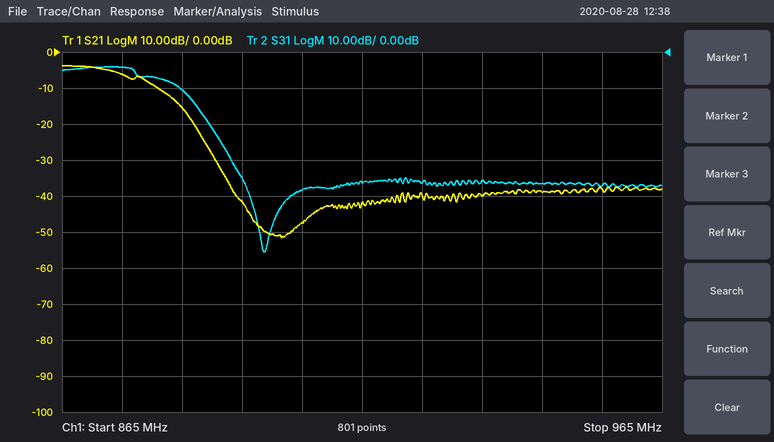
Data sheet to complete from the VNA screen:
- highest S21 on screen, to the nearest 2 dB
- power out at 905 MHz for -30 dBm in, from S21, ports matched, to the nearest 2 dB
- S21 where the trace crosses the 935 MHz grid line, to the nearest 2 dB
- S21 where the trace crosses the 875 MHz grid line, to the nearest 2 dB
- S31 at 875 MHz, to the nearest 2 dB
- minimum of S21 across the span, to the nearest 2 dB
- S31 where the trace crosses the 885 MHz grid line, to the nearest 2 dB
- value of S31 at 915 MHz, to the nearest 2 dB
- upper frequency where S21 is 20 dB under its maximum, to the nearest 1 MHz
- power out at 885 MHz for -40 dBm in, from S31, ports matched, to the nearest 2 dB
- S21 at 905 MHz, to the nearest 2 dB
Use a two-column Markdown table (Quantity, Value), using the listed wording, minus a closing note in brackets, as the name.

| Quantity | Value |
|---|---|
| highest S21 on screen, to the nearest 2 dB | -4 dB |
| power out at 905 MHz for -30 dBm in, from S21, ports matched, to the nearest 2 dB | -78 dBm |
| S21 where the trace crosses the 935 MHz grid line, to the nearest 2 dB | -40 dB |
| S21 where the trace crosses the 875 MHz grid line, to the nearest 2 dB | -6 dB |
| S31 at 875 MHz, to the nearest 2 dB | -4 dB |
| minimum of S21 across the span, to the nearest 2 dB | -52 dB |
| S31 where the trace crosses the 885 MHz grid line, to the nearest 2 dB | -10 dB |
| value of S31 at 915 MHz, to the nearest 2 dB | -36 dB |
| upper frequency where S21 is 20 dB under its maximum, to the nearest 1 MHz | 888 MHz |
| power out at 885 MHz for -40 dBm in, from S31, ports matched, to the nearest 2 dB | -50 dBm |
| S21 at 905 MHz, to the nearest 2 dB | -48 dB |
